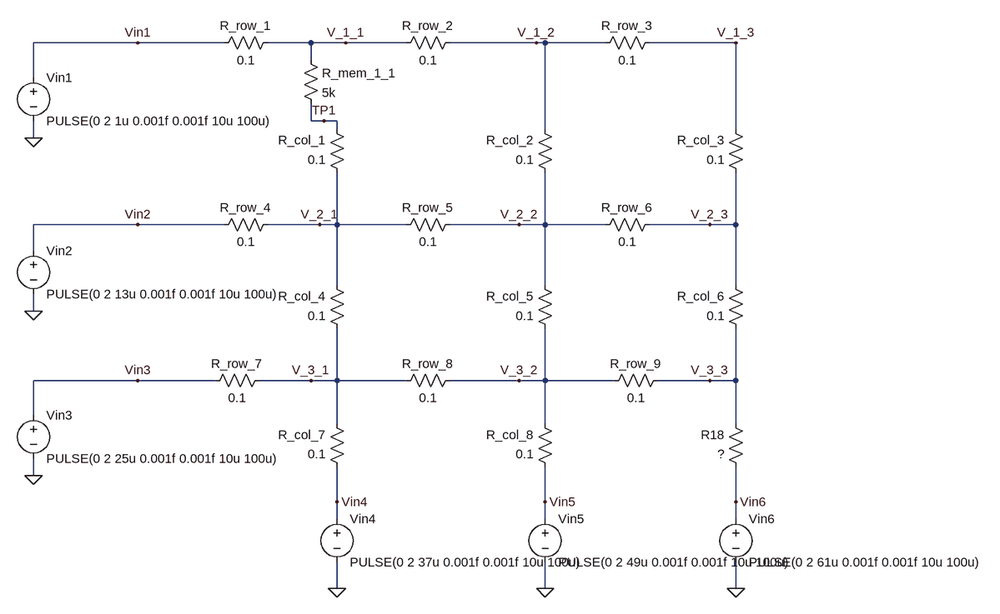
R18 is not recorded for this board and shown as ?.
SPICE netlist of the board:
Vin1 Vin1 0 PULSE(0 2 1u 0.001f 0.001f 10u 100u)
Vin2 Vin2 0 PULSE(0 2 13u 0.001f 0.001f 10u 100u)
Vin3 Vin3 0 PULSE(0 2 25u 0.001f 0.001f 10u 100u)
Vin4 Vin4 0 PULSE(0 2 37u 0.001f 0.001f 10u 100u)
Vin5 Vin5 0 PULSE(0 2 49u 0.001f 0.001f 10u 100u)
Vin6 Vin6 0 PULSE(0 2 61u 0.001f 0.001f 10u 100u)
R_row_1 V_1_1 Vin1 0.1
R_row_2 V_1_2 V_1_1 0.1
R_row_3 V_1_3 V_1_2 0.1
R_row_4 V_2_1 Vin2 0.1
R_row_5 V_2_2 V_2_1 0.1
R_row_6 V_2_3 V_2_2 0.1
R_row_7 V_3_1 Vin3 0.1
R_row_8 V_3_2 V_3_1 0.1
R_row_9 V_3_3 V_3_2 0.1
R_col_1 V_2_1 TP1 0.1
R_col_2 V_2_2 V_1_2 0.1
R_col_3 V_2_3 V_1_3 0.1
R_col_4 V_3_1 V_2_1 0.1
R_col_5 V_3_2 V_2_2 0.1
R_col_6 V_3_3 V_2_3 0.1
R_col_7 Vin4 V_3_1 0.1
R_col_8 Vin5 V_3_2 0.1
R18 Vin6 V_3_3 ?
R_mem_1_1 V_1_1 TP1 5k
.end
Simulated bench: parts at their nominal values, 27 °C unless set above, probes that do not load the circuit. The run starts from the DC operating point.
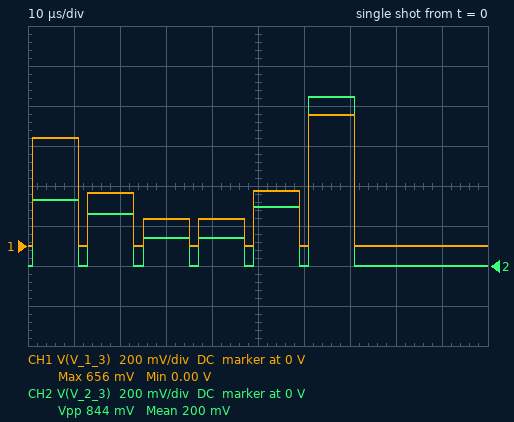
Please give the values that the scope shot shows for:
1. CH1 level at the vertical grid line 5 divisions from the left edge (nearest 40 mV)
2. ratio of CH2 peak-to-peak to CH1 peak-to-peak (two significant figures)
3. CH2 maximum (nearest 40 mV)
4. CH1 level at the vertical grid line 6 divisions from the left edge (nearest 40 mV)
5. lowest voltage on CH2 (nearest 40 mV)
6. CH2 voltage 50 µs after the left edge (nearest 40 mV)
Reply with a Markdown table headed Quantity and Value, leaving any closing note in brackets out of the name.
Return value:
| Quantity | Value |
|---|---|
| CH1 level at the vertical grid line 5 divisions from the left edge | 280 mV |
| ratio of CH2 peak-to-peak to CH1 peak-to-peak | 1.3 |
| CH2 maximum | 840 mV |
| CH1 level at the vertical grid line 6 divisions from the left edge | 0 V |
| lowest voltage on CH2 | 0 V |
| CH2 voltage 50 µs after the left edge | 280 mV |
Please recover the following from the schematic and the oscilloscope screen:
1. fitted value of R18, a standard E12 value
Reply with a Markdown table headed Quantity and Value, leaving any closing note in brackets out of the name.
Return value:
| Quantity | Value |
|---|---|
| fitted value of R18, a standard E12 value | 0.047 Ω |
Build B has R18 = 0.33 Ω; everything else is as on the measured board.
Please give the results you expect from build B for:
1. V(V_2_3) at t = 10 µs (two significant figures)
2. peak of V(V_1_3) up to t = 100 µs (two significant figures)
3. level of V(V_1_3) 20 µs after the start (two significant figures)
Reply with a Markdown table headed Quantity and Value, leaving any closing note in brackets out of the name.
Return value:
| Quantity | Value |
|---|---|
| V(V_2_3) at t = 10 µs | 420 mV |
| peak of V(V_1_3) up to t = 100 µs | 610 mV |
| level of V(V_1_3) 20 µs after the start | 340 mV |
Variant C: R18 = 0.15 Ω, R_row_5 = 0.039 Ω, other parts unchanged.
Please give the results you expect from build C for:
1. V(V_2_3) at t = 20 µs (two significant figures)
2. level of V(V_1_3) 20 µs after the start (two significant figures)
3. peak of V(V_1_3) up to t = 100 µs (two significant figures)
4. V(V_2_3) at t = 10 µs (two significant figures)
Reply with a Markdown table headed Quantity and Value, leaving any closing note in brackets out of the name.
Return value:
| Quantity | Value |
|---|---|
| V(V_2_3) at t = 20 µs | 410 mV |
| level of V(V_1_3) 20 µs after the start | 400 mV |
| peak of V(V_1_3) up to t = 100 µs | 540 mV |
| V(V_2_3) at t = 10 µs | 350 mV |
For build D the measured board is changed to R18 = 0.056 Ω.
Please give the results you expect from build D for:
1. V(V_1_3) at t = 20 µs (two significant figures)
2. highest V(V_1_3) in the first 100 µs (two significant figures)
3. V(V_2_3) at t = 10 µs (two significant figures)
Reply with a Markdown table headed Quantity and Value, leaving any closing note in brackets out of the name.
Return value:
| Quantity | Value |
|---|---|
| V(V_1_3) at t = 20 µs | 270 mV |
| highest V(V_1_3) in the first 100 µs | 620 mV |
| V(V_2_3) at t = 10 µs | 340 mV |
